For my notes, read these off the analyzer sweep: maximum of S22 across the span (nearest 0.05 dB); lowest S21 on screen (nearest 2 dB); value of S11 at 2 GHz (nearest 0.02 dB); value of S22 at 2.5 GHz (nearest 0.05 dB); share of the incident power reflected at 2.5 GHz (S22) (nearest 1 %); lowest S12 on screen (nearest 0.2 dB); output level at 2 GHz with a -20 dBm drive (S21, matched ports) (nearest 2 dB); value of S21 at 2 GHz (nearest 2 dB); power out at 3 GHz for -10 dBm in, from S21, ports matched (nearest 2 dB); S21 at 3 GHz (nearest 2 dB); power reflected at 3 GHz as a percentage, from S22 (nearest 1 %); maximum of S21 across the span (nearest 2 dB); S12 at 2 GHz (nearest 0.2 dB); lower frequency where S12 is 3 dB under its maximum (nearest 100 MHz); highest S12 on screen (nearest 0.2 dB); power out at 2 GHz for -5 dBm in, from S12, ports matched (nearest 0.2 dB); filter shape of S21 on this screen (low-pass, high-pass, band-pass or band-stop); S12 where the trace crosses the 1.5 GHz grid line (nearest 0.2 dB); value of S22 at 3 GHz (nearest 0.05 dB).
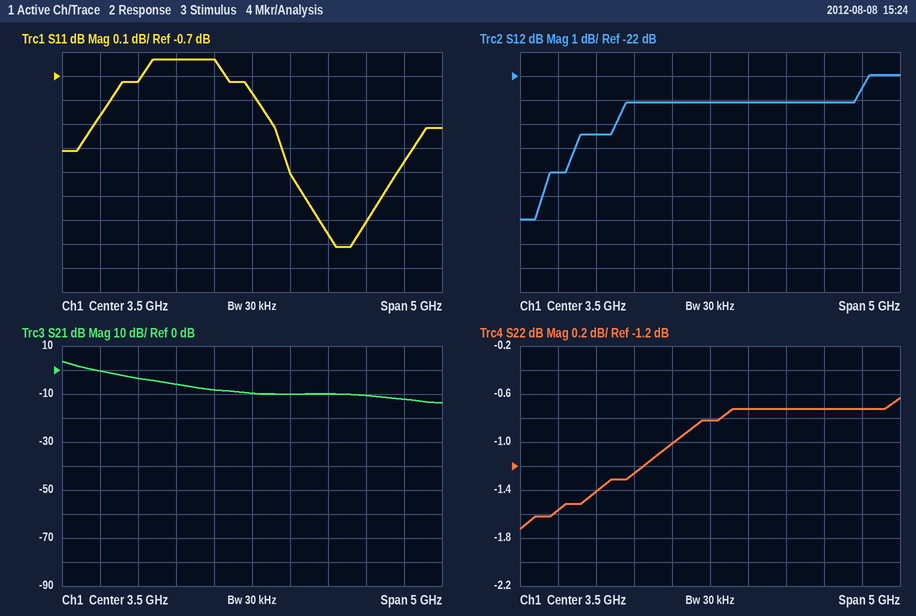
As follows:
-0.65 dB
-14 dB
-0.72 dB
-1.25 dB
75 %
-28.0 dB
-24 dBm
-4 dB
-18 dBm
-8 dB
79 %
4 dB
-24.4 dB
1.7 GHz
-22.0 dB
-29.4 dBm
low-pass
-26.0 dB
-1.00 dB
